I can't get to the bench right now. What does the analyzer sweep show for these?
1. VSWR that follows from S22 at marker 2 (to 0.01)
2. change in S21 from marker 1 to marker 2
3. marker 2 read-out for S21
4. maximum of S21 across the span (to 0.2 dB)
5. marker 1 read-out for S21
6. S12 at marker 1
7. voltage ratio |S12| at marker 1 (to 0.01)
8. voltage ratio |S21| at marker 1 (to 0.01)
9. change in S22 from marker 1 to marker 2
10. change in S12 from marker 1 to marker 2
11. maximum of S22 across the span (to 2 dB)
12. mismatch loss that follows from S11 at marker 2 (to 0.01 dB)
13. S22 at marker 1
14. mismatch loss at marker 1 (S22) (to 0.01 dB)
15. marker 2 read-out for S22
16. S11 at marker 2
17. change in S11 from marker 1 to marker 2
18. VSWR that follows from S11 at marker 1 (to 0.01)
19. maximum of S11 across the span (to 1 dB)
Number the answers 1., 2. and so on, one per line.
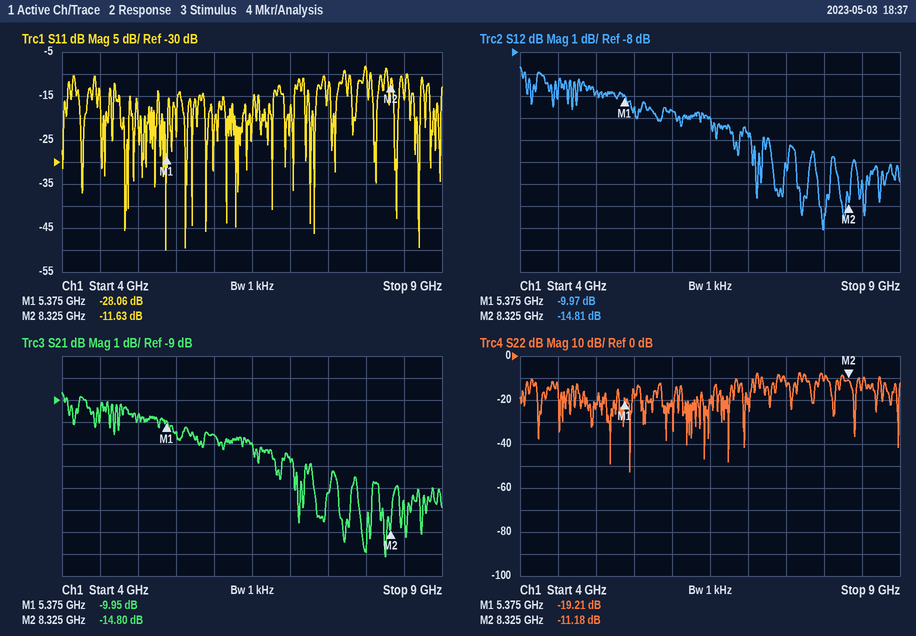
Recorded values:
1. 1.76
2. -4.85 dB
3. -14.80 dB
4. -8.6 dB
5. -9.95 dB
6. -9.97 dB
7. 0.32
8. 0.32
9. 8.03 dB
10. -4.84 dB
11. -8 dB
12. 0.31 dB
13. -19.21 dB
14. 0.05 dB
15. -11.18 dB
16. -11.63 dB
17. 16.43 dB
18. 1.08
19. -8 dB
